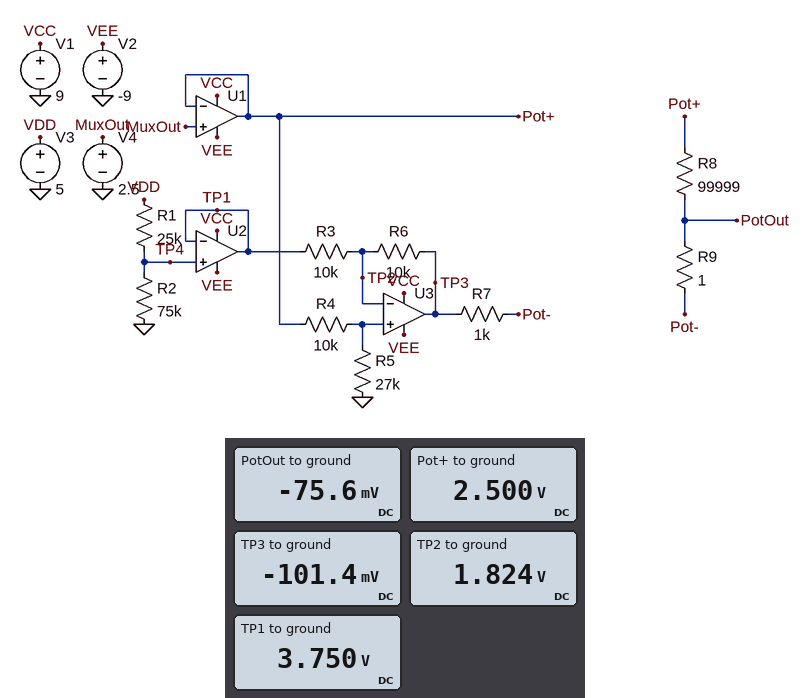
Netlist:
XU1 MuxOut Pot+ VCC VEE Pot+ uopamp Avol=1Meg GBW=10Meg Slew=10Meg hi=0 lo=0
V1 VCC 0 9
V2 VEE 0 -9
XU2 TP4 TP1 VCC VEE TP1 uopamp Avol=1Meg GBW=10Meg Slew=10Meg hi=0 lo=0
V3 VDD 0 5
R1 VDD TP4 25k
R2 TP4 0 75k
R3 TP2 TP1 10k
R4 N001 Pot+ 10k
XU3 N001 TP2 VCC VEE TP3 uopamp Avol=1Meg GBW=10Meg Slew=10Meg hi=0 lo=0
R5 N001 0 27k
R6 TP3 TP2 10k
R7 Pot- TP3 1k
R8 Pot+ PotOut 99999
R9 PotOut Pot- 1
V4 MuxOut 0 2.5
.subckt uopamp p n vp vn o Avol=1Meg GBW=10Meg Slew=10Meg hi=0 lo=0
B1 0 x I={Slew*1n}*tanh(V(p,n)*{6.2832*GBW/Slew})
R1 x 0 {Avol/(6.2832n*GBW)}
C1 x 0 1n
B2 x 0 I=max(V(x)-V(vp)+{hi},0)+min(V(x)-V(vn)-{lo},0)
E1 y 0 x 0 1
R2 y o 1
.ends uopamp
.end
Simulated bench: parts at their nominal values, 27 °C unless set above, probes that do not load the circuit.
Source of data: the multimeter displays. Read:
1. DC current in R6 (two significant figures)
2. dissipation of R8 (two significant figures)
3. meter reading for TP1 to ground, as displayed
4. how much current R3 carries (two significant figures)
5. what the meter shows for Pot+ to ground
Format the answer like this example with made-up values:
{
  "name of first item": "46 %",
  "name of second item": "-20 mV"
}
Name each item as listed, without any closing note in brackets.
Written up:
{
  "DC current in R6": "190 µA",
  "dissipation of R8": "66 µW",
  "meter reading for TP1 to ground, as displayed": "3.750 V",
  "how much current R3 carries": "190 µA",
  "what the meter shows for Pot+ to ground": "2.500 V"
}
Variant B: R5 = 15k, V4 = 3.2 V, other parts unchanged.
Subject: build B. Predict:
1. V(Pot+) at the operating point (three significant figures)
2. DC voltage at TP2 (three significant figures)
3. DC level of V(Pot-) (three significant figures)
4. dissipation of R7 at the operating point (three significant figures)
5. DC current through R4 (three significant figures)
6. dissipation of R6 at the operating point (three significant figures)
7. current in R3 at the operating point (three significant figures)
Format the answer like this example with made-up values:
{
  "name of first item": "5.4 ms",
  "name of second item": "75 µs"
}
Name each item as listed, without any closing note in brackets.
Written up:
{
  "V(Pot+) at the operating point": "3.20 V",
  "DC voltage at TP2": "1.92 V",
  "DC level of V(Pot-)": "121 mV",
  "dissipation of R7 at the operating point": "948 nW",
  "DC current through R4": "128 µA",
  "dissipation of R6 at the operating point": "335 µW",
  "current in R3 at the operating point": "183 µA"
}
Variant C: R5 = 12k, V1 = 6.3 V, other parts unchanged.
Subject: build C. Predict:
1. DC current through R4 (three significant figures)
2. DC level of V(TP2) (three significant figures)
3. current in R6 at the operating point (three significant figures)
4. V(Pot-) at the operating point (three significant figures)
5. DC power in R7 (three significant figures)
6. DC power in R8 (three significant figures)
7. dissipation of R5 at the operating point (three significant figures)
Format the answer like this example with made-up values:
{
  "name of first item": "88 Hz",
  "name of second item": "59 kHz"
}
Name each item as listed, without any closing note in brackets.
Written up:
{
  "DC current through R4": "114 µA",
  "DC level of V(TP2)": "1.36 V",
  "current in R6 at the operating point": "239 µA",
  "V(Pot-) at the operating point": "-988 mV",
  "DC power in R7": "1.22 µW",
  "DC power in R8": "122 µW",
  "dissipation of R5 at the operating point": "155 µW"
}
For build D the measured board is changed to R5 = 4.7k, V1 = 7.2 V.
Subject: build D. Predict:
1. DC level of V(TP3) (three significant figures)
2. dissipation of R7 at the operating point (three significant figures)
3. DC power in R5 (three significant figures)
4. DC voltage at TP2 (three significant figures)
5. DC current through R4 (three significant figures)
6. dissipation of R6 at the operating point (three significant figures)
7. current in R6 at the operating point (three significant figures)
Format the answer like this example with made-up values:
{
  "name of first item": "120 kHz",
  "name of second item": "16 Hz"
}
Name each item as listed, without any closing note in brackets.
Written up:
{
  "DC level of V(TP3)": "-2.15 V",
  "dissipation of R7 at the operating point": "2.12 µW",
  "DC power in R5": "136 µW",
  "DC voltage at TP2": "799 mV",
  "DC current through R4": "170 µA",
  "dissipation of R6 at the operating point": "871 µW",
  "current in R6 at the operating point": "295 µA"
}
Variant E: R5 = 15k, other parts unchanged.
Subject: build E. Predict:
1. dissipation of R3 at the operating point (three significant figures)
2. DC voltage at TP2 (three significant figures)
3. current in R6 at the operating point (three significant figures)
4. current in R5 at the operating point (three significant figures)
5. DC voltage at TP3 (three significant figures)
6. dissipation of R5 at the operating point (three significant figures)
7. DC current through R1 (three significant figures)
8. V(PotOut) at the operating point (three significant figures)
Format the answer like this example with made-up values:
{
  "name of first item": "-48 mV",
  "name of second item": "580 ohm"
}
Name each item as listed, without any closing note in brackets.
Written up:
{
  "dissipation of R3 at the operating point": "506 µW",
  "DC voltage at TP2": "1.50 V",
  "current in R6 at the operating point": "225 µA",
  "current in R5 at the operating point": "100 µA",
  "DC voltage at TP3": "-750 mV",
  "dissipation of R5 at the operating point": "150 µW",
  "DC current through R1": "50.0 µA",
  "V(PotOut) at the operating point": "-718 mV"
}
